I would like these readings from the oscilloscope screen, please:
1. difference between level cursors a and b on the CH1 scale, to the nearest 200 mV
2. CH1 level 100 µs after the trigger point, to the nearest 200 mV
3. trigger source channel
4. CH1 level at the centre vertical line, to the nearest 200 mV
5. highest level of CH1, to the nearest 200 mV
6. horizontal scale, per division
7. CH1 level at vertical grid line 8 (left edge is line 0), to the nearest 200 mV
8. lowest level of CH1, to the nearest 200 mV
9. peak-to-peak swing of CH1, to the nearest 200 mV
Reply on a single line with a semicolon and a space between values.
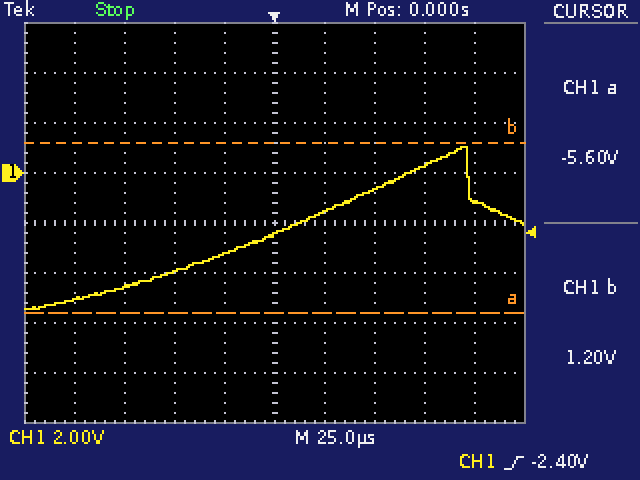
6.8 V; -1.2 V; CH1; -2.4 V; 1.0 V; 25 µs; 400 mV; -5.4 V; 6.4 V
